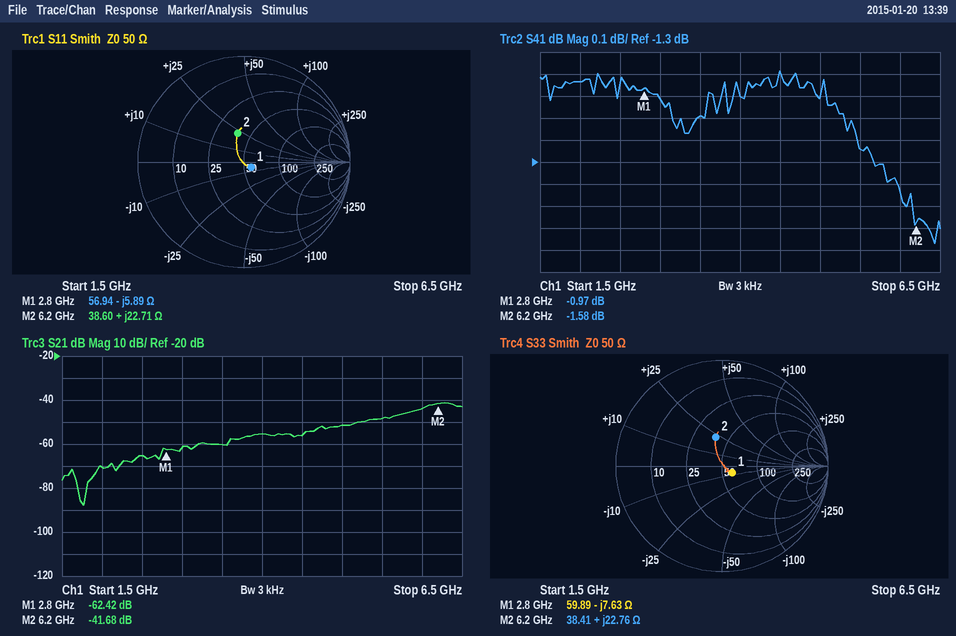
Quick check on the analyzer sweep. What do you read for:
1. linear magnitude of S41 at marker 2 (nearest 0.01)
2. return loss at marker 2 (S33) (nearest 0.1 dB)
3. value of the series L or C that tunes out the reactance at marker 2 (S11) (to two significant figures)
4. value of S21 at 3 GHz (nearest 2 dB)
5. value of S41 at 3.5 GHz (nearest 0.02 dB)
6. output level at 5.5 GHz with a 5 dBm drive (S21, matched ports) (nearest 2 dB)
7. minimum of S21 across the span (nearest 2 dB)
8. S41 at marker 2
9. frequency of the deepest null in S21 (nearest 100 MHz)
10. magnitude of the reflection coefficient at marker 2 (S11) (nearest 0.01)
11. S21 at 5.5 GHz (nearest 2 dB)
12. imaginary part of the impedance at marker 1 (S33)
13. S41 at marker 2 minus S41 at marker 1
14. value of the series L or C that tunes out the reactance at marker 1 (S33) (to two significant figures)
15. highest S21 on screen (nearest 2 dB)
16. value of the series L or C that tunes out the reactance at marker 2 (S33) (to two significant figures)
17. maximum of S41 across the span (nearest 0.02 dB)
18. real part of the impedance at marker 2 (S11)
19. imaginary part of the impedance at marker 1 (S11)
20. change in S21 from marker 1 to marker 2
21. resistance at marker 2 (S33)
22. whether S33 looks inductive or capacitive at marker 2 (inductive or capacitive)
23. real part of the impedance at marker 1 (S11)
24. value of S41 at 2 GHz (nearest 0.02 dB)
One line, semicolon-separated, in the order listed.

0.83; 11.1 dB; 1.1 pF; -62 dB; -1.10 dB; -44 dBm; -88 dB; -1.58 dB; 1.8 GHz; 0.28; -48 dB; -7.63 Ω; -0.61 dB; 430 pH; -42 dB; 1.1 pF; -0.88 dB; 38.60 Ω; -5.89 Ω; 20.74 dB; 38.41 Ω; inductive; 56.94 Ω; -0.94 dB
